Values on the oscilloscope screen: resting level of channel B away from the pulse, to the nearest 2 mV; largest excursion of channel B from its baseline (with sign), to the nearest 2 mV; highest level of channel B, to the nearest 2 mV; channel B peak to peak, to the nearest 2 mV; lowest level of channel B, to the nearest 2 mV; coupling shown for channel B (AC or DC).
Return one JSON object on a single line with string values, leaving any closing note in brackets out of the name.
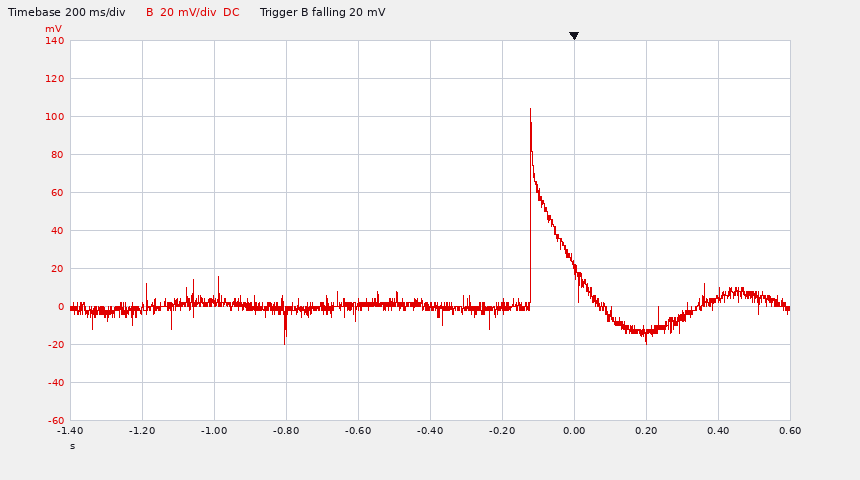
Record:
{"resting level of channel B away from the pulse, to the nearest 2 mV": "0 mV", "largest excursion of channel B from its baseline (with sign), to the nearest 2 mV": "+104 mV", "highest level of channel B, to the nearest 2 mV": "104 mV", "channel B peak to peak, to the nearest 2 mV": "124 mV", "lowest level of channel B, to the nearest 2 mV": "-20 mV", "coupling shown for channel B": "DC"}
